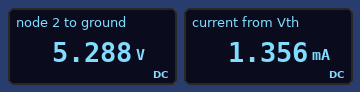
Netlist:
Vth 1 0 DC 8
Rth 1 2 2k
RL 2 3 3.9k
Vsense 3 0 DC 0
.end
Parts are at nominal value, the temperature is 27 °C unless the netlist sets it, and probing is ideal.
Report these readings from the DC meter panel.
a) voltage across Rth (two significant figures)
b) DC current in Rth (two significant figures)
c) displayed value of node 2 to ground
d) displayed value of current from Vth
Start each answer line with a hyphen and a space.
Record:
- 2.7 V
- 1.4 mA
- 5.288 V
- 1.356 mA
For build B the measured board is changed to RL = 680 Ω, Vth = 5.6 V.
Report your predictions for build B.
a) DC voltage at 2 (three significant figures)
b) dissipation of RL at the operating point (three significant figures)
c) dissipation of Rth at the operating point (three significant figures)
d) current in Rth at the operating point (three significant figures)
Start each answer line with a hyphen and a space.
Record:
- 1.42 V
- 2.97 mW
- 8.73 mW
- 2.09 mA
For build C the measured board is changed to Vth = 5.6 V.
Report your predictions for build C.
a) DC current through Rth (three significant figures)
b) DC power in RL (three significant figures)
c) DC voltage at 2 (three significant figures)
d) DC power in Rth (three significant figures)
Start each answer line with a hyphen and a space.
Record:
- 949 µA
- 3.51 mW
- 3.70 V
- 1.80 mW
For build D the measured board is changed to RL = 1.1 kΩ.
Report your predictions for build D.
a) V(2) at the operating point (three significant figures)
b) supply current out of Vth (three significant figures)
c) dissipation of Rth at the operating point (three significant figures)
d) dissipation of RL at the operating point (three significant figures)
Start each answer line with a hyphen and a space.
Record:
- 2.84 V
- 2.58 mA
- 13.3 mW
- 7.33 mW
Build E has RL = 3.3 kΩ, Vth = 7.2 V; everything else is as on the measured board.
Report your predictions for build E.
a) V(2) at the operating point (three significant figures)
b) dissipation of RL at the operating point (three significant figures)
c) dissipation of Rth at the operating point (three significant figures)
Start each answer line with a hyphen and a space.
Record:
- 4.48 V
- 6.09 mW
- 3.69 mW
